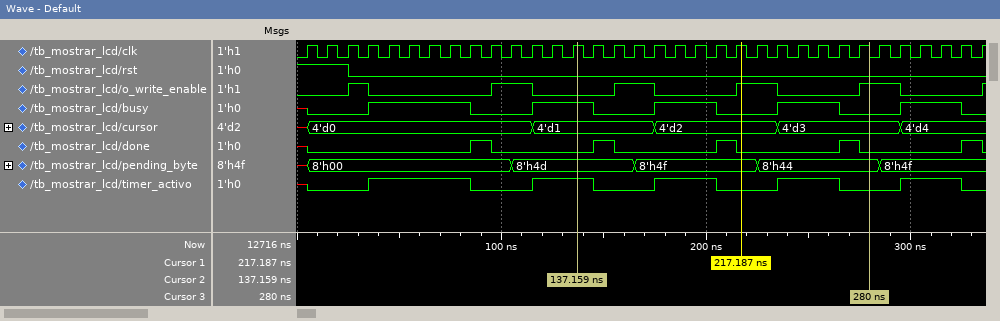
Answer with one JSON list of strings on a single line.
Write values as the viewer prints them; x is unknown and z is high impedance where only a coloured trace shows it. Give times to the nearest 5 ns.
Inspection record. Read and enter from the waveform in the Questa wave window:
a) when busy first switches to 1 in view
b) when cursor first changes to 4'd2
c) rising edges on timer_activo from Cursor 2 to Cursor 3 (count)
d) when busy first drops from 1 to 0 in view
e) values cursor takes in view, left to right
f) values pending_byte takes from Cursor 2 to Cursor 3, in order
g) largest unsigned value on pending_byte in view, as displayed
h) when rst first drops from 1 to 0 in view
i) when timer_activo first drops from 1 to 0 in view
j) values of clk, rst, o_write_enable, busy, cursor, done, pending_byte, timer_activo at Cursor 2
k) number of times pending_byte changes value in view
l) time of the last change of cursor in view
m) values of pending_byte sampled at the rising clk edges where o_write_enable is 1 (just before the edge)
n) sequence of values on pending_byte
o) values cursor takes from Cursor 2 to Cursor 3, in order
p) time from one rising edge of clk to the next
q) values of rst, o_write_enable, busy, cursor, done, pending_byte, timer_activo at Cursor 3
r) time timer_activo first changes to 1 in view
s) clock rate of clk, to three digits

["35 ns", "175 ns", "2", "85 ns", "x, 4'd0, 4'd1, 4'd2, 4'd3, 4'd4", "8'h4d, 8'h4f, 8'h44", "8'h4f", "25 ns", "85 ns", "clk=1, rst=0, o_write_enable=0, busy=1, cursor=4'd1, done=0, pending_byte=8'h4d, timer_activo=1", "5", "295 ns", "8'h00, 8'h00, 8'h4d, 8'h4d, 8'h4f, 8'h4f, 8'h44, 8'h44, 8'h4f", "x, 8'h00, 8'h4d, 8'h4f, 8'h44, 8'h4f", "4'd1, 4'd2, 4'd3", "10 ns", "rst=0, o_write_enable=1, busy=0, cursor=4'd3, done=0, pending_byte=8'h44, timer_activo=0", "35 ns", "100 MHz"]
